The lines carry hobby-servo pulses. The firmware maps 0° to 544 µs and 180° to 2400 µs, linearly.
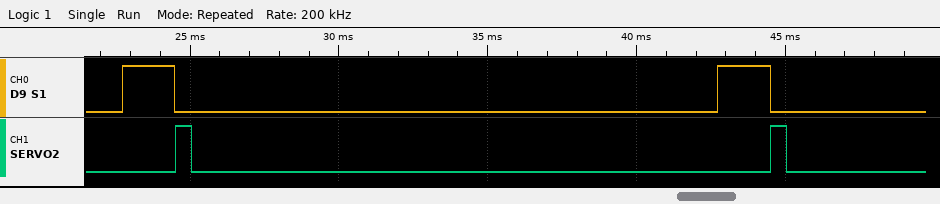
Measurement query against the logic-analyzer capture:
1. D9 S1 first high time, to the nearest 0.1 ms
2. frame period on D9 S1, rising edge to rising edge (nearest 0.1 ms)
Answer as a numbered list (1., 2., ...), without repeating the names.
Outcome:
1. 1.8 ms
2. 20.0 ms
